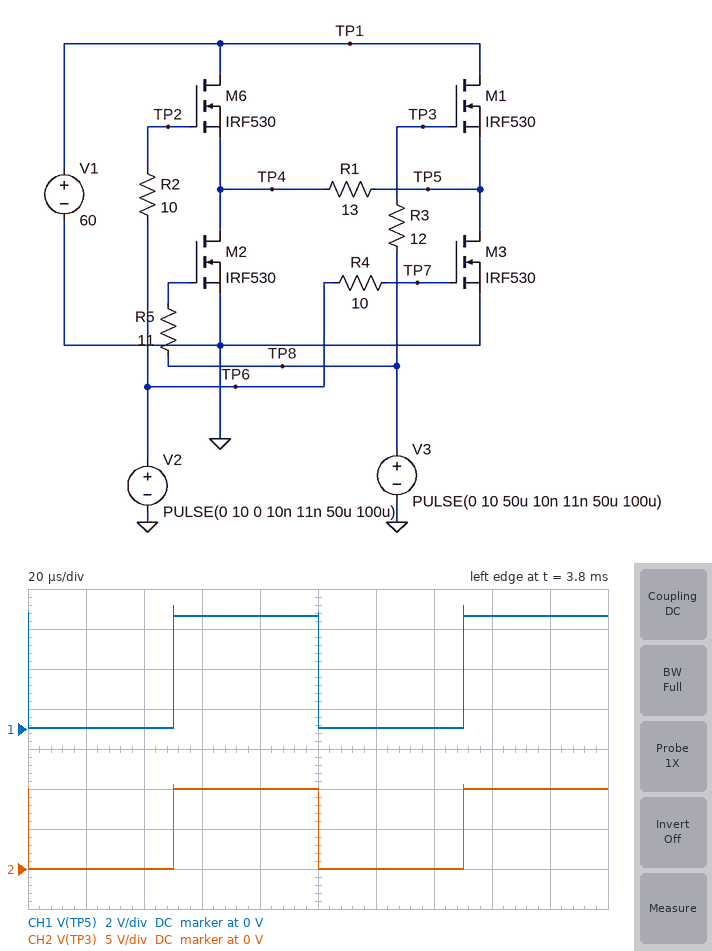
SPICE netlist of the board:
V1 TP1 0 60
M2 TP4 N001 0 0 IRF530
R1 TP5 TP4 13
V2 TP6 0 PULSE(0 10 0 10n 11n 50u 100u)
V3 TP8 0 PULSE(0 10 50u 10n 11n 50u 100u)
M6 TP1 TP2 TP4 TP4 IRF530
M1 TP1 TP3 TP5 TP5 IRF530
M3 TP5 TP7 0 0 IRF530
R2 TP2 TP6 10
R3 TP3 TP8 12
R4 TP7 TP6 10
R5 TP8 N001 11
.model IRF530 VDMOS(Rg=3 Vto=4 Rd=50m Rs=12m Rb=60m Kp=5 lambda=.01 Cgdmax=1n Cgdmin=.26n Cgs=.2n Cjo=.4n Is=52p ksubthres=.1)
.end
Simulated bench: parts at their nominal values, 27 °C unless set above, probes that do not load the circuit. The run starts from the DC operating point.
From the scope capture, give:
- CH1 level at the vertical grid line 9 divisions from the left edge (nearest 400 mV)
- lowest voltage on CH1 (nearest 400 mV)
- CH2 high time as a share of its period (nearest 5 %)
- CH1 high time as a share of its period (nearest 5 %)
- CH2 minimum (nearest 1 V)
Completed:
5.6 V
0 V
50 %
50 %
0 V
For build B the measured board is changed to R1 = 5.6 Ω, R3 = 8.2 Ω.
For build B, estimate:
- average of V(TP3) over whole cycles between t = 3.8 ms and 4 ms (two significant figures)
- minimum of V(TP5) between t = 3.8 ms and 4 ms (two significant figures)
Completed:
5.0 V
92 mV
